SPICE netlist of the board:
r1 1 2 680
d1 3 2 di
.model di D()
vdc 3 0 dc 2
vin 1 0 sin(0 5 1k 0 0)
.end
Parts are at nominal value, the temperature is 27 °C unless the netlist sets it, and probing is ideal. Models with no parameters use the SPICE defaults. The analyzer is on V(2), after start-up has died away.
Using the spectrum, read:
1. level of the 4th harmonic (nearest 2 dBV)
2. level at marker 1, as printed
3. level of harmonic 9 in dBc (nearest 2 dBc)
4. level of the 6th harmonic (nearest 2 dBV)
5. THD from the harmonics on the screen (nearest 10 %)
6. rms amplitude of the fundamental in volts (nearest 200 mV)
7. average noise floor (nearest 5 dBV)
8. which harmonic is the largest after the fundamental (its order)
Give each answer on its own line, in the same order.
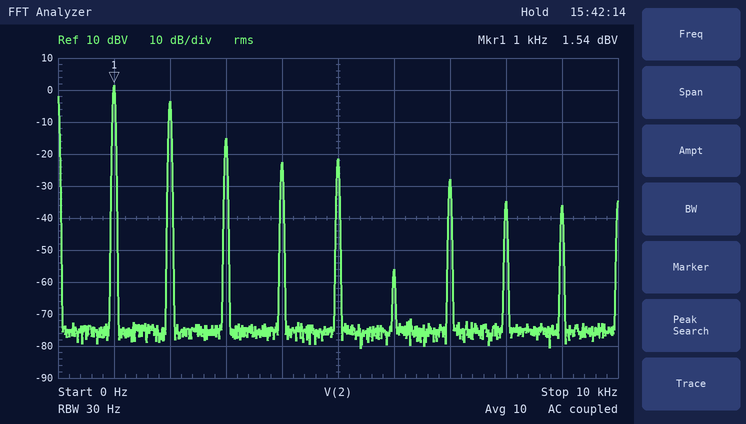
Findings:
-22 dBV
1.54 dBV
-38 dBc
-56 dBV
60 %
1.2 V
-75 dBV
2
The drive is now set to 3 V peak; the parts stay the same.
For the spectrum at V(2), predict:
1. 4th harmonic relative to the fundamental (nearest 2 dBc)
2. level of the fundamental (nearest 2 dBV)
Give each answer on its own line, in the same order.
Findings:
-32 dBc
-6 dBV
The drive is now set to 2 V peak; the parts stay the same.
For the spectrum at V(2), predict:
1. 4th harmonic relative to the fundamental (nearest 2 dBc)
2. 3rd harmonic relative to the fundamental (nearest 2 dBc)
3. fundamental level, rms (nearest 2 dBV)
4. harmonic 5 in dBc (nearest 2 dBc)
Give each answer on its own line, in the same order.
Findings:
-14 dBc
-8 dBc
-16 dBV
-24 dBc
